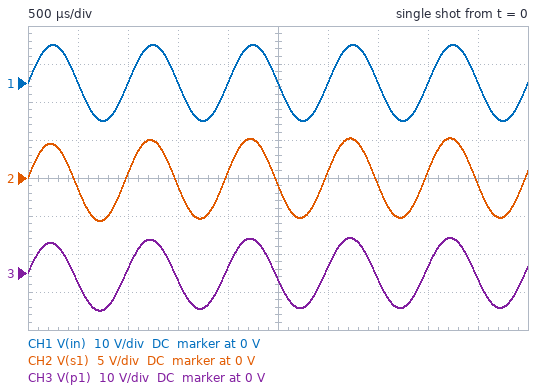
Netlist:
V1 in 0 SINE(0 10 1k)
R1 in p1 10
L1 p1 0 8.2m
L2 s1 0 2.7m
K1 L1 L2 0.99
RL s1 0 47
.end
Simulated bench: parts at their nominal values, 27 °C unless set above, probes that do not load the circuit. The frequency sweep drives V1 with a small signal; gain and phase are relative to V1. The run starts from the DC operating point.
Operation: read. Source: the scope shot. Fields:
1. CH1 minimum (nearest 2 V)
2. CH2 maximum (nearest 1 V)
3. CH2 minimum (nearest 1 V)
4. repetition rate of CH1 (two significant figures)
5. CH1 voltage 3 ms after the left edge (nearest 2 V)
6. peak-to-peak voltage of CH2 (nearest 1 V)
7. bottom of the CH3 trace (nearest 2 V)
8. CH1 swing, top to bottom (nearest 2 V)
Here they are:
-10 V
5 V
-6 V
1.0 kHz
0 V
11 V
-10 V
20 V
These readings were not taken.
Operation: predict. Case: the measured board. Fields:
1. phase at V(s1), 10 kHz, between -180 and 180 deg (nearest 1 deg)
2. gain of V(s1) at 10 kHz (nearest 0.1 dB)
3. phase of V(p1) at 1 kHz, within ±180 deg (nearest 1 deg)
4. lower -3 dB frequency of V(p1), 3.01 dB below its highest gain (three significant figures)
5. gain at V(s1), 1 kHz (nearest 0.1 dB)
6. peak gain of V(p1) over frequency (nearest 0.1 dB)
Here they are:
-3 deg
-5.5 dB
10 deg
210 Hz
-5.6 dB
0 dB
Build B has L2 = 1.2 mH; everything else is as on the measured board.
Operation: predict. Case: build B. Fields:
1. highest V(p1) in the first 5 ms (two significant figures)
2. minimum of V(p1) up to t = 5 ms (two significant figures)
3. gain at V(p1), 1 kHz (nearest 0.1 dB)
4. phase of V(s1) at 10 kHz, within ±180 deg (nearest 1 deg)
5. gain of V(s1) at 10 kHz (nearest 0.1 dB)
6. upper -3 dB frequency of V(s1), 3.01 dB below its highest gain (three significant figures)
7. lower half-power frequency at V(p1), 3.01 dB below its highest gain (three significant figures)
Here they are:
9.5 V
-10 V
-0.4 dB
-1 deg
-8.7 dB
323 kHz
200 Hz
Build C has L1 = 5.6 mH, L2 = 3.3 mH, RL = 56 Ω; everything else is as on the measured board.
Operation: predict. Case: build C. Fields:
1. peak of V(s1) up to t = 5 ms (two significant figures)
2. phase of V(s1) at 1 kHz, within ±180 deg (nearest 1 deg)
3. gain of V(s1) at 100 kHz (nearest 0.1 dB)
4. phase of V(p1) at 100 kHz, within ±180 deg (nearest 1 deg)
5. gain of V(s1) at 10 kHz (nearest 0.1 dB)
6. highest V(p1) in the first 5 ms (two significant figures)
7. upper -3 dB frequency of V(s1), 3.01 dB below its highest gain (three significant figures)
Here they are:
6.7 V
14 deg
-4.8 dB
3 deg
-3.3 dB
8.8 V
150 kHz
